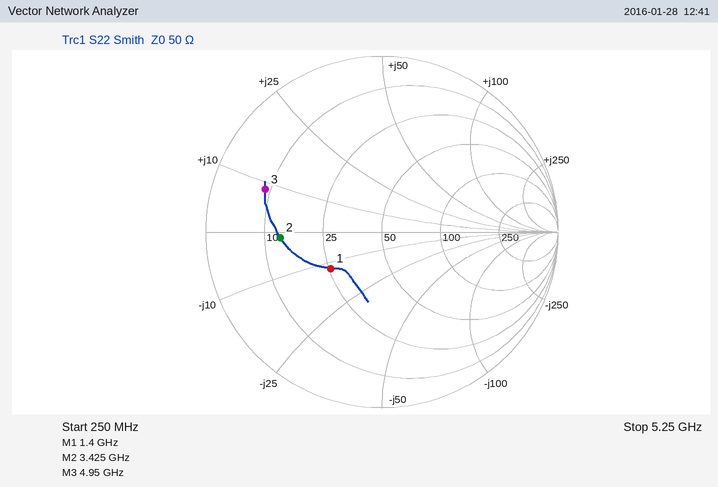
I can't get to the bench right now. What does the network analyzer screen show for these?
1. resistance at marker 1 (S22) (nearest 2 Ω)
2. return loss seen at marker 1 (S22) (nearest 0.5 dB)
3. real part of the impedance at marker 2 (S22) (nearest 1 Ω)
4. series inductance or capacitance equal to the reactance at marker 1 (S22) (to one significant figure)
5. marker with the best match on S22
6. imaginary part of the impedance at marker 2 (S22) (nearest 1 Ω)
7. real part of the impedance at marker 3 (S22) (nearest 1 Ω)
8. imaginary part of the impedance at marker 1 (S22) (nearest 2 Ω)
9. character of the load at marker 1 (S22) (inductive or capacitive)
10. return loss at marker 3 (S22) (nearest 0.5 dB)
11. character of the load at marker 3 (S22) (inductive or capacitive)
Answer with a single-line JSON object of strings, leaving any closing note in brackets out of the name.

{"resistance at marker 1 (S22)": "26 Ω", "return loss seen at marker 1 (S22)": "9.0 dB", "real part of the impedance at marker 2 (S22)": "13 Ω", "series inductance or capacitance equal to the reactance at marker 1 (S22)": "9 pF", "marker with the best match on S22": "marker 1", "imaginary part of the impedance at marker 2 (S22)": "-1 Ω", "real part of the impedance at marker 3 (S22)": "9 Ω", "imaginary part of the impedance at marker 1 (S22)": "-12 Ω", "character of the load at marker 1 (S22)": "capacitive", "return loss at marker 3 (S22)": "3.0 dB", "character of the load at marker 3 (S22)": "inductive"}
